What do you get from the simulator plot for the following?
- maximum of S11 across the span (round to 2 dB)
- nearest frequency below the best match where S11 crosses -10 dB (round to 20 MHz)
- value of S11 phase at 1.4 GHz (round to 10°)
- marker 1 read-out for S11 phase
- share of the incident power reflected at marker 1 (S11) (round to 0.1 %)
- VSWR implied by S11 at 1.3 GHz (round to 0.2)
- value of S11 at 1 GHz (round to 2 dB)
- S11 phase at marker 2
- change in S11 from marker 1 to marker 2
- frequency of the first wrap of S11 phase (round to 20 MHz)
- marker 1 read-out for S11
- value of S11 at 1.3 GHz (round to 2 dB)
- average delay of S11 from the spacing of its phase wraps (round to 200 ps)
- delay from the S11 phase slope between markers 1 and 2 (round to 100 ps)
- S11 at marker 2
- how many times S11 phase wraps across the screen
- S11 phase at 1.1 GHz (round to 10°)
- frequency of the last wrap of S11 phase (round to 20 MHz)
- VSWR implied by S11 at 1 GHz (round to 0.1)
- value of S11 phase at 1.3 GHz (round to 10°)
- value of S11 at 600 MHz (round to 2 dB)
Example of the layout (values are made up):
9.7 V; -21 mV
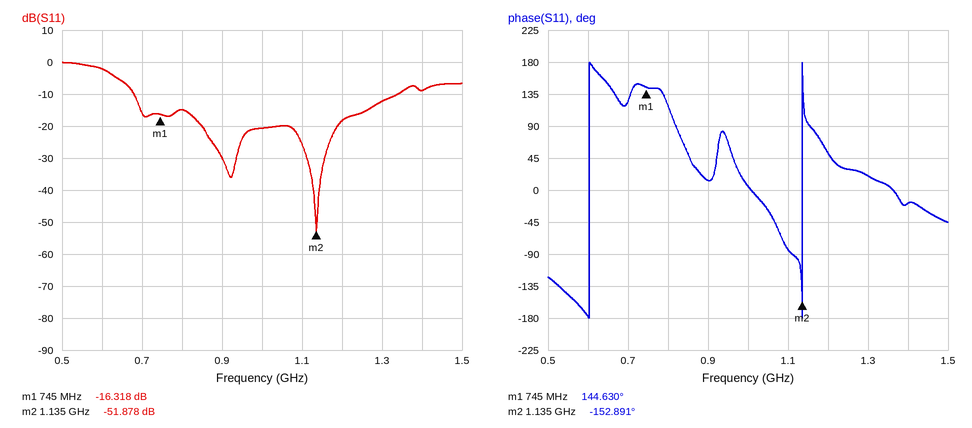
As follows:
0 dB; 680 MHz; -20°; 144.630°; 2.3 %; 1.6; -20 dB; -152.891°; -35.560 dB; 600 MHz; -16.318 dB; -12 dB; 1.8 ns; 2.1 ns; -51.878 dB; 2; -80°; 1.14 GHz; 1.2; 20°; -2 dB
